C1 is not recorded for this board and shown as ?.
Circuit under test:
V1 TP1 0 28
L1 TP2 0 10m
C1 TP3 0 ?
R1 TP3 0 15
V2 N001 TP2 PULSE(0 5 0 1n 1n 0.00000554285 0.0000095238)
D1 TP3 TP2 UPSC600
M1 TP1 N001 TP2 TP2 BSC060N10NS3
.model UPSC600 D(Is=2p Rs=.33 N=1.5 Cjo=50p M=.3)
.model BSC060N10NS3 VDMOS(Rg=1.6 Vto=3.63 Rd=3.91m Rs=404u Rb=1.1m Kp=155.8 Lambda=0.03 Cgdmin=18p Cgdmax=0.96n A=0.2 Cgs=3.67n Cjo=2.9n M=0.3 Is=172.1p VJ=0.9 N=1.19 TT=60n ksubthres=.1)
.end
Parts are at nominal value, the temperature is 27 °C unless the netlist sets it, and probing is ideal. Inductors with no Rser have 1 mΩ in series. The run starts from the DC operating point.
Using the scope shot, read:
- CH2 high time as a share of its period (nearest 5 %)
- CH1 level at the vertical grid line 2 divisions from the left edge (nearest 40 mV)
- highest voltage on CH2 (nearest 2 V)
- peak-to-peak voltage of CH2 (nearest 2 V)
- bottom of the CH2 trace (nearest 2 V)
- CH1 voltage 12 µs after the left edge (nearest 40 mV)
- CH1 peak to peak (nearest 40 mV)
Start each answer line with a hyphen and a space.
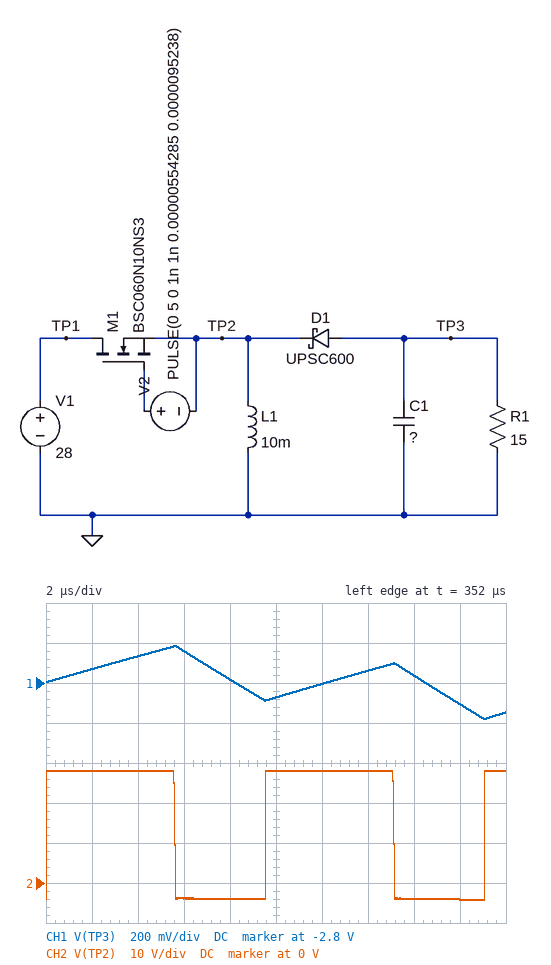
- 60 %
- -2.68 V
- 28 V
- 32 V
- -4 V
- -2.80 V
- 360 mV
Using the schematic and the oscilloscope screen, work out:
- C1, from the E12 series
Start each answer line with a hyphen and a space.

- 5.6 µF
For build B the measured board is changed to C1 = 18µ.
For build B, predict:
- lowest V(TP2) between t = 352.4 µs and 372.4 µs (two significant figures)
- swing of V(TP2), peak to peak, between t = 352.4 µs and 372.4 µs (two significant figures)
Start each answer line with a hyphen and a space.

- -3.0 V
- 31 V
